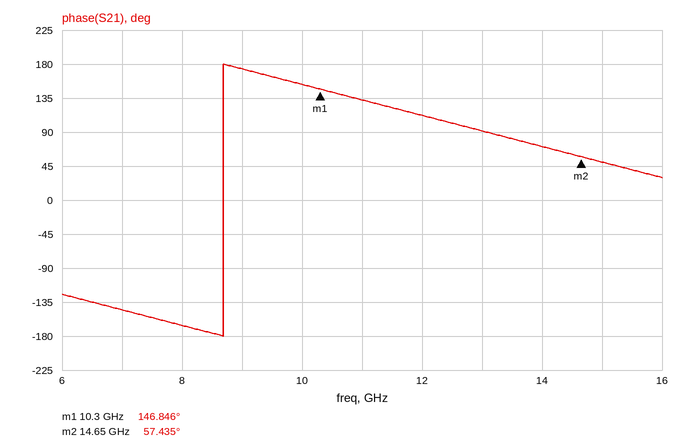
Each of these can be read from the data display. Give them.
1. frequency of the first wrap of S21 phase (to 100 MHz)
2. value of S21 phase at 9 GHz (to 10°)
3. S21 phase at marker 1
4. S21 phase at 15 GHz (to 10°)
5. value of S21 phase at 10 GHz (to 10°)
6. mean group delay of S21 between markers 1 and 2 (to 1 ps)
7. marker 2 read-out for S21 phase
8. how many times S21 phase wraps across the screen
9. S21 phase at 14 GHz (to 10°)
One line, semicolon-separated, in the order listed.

8.7 GHz; 170°; 146.846°; 50°; 150°; 57 ps; 57.435°; 1; 70°
